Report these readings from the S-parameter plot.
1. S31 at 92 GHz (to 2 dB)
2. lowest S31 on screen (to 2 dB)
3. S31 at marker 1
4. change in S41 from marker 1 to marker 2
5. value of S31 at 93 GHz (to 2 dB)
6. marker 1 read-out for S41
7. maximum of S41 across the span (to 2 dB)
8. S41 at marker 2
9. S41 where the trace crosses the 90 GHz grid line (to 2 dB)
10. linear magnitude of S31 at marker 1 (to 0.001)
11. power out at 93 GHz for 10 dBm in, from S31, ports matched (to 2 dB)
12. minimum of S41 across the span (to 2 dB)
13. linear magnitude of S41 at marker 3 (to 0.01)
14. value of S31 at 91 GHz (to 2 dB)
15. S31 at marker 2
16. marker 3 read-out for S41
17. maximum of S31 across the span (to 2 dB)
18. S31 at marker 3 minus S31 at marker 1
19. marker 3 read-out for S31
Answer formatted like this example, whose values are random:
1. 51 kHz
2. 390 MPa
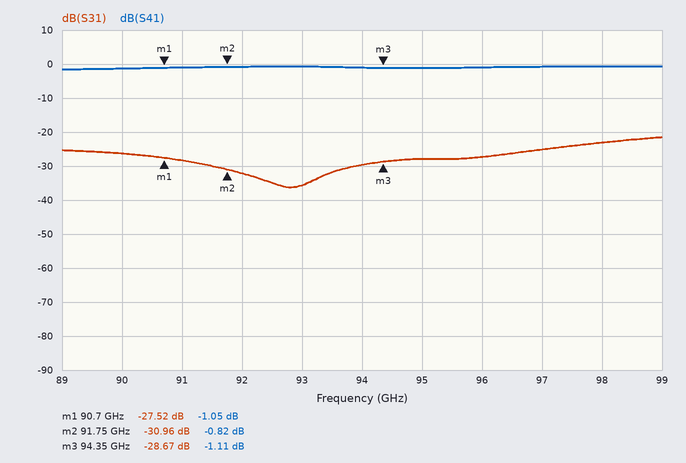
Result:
1. -32 dB
2. -36 dB
3. -27.52 dB
4. 0.23 dB
5. -36 dB
6. -1.05 dB
7. 0 dB
8. -0.82 dB
9. -2 dB
10. 0.042
11. -26 dBm
12. -2 dB
13. 0.88
14. -28 dB
15. -30.96 dB
16. -1.11 dB
17. -22 dB
18. -1.15 dB
19. -28.67 dB
